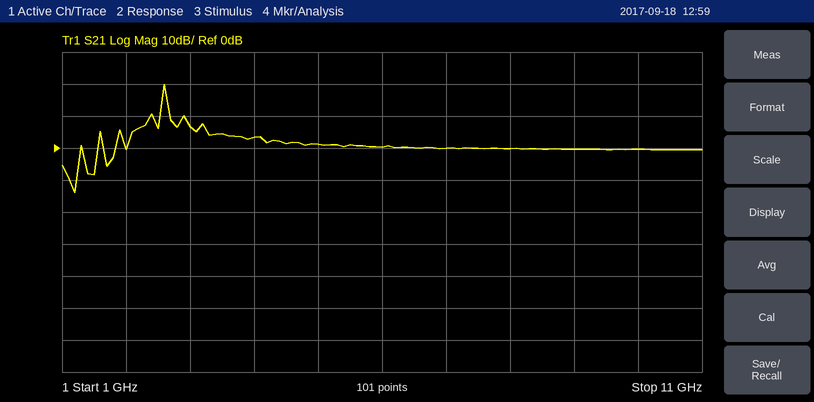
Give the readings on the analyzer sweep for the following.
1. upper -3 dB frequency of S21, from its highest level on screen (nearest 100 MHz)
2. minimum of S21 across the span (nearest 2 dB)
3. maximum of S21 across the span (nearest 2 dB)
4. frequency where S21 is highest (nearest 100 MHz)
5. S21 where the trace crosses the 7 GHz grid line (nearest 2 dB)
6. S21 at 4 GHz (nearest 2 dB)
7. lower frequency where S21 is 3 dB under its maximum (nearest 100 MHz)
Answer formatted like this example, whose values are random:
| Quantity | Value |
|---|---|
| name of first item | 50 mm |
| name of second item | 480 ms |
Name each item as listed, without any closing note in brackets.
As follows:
| Quantity | Value |
|---|---|
| upper -3 dB frequency of S21, from its highest level on screen | 2.6 GHz |
| minimum of S21 across the span | -14 dB |
| maximum of S21 across the span | 20 dB |
| frequency where S21 is highest | 2.6 GHz |
| S21 where the trace crosses the 7 GHz grid line | 0 dB |
| S21 at 4 GHz | 4 dB |
| lower frequency where S21 is 3 dB under its maximum | 2.6 GHz |
